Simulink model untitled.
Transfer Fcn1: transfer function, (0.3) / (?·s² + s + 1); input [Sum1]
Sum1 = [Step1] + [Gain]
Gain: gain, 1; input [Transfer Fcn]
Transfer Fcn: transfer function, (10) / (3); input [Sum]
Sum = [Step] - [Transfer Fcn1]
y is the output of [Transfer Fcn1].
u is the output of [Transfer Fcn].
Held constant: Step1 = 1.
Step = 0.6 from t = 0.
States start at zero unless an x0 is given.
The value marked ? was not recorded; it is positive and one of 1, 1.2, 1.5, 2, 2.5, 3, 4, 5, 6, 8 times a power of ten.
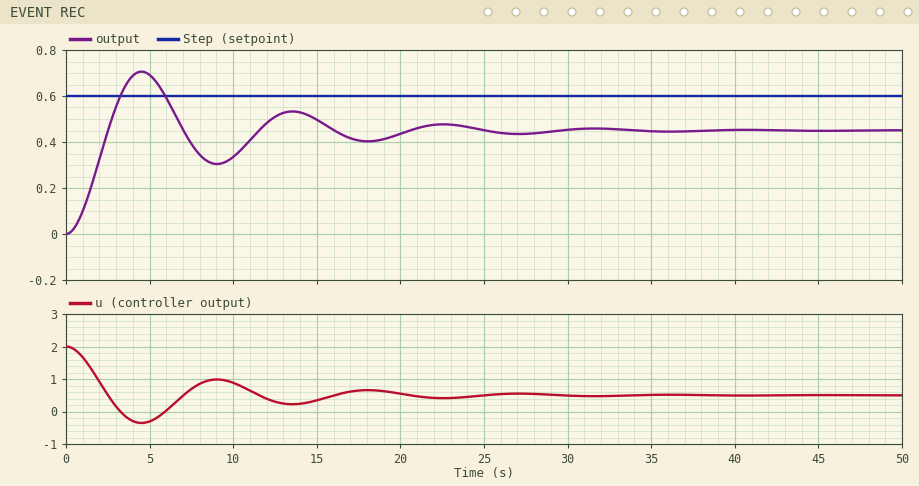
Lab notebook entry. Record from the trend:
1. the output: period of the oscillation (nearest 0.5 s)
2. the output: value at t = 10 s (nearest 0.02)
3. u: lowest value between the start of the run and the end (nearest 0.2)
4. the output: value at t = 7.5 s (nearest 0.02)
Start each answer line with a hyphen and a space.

- 9.0 s
- 0.34
- -0.4
- 0.40
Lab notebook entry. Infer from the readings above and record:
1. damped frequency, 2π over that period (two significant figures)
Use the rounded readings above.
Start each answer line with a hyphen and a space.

- 0.70 rad/s
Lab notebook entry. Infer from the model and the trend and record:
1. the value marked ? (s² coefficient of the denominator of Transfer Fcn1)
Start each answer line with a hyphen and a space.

- 4
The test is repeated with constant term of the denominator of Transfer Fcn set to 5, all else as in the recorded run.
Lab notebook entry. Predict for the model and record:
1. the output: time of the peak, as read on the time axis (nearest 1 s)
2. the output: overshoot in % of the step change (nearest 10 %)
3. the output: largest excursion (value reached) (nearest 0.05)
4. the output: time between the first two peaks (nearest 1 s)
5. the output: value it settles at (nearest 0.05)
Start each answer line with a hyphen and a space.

- 5 s
- 50 %
- 0.65
- 10 s
- 0.40
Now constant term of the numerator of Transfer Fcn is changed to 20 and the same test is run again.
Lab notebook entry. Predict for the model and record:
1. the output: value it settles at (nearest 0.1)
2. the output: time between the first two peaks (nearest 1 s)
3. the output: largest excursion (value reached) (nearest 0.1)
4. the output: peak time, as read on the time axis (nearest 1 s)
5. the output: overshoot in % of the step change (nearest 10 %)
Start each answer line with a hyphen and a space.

- 0.5
- 7 s
- 0.8
- 4 s
- 60 %
